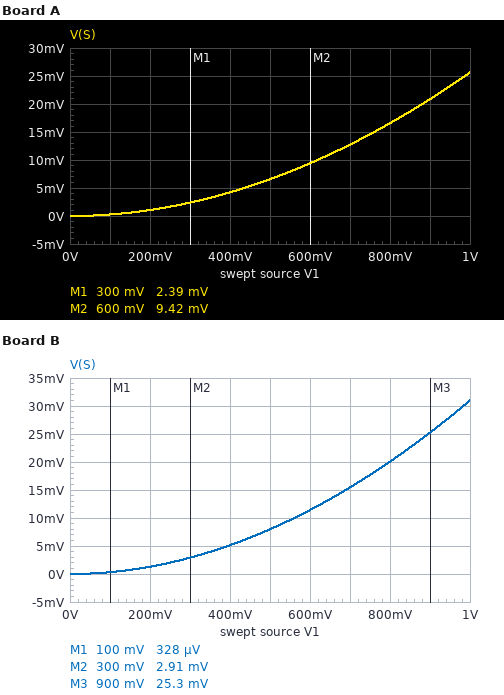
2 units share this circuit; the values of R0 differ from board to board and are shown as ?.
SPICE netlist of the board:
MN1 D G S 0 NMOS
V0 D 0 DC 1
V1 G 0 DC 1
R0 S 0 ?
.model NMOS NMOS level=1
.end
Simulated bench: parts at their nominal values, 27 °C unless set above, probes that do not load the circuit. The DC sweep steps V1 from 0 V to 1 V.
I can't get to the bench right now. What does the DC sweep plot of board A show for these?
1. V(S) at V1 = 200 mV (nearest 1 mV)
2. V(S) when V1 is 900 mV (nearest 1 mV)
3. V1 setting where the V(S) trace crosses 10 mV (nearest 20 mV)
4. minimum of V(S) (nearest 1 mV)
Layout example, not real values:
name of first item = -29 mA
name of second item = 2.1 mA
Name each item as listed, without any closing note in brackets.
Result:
V(S) at V1 = 200 mV = 1 mV
V(S) when V1 is 900 mV = 21 mV
V1 setting where the V(S) trace crosses 10 mV = 620 mV
minimum of V(S) = 0 V
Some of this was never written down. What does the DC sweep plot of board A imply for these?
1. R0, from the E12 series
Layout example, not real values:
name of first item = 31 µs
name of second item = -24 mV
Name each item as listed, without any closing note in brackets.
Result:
R0, from the E12 series = 2.7 kΩ
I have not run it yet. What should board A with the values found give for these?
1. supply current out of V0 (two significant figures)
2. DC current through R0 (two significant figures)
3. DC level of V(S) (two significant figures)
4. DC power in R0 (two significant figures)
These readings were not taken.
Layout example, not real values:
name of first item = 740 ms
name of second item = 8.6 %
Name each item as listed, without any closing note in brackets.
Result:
supply current out of V0 = 9.5 µA
DC current through R0 = 9.5 µA
DC level of V(S) = 26 mV
DC power in R0 = 240 nW
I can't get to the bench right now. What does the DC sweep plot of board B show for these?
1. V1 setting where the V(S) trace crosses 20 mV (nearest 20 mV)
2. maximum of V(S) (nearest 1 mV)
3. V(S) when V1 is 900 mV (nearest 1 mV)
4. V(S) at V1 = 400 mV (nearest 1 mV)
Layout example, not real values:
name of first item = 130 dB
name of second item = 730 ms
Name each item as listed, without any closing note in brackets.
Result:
V1 setting where the V(S) trace crosses 20 mV = 800 mV
maximum of V(S) = 31 mV
V(S) when V1 is 900 mV = 25 mV
V(S) at V1 = 400 mV = 5 mV
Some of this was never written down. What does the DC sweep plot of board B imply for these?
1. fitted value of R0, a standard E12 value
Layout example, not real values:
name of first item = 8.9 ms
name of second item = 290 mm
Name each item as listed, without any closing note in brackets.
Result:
fitted value of R0, a standard E12 value = 3.3 kΩ
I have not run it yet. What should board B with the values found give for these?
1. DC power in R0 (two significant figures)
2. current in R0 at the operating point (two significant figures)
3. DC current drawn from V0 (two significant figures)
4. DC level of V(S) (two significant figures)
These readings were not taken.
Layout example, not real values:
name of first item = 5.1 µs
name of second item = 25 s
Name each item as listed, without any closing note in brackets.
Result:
DC power in R0 = 290 nW
current in R0 at the operating point = 9.4 µA
DC current drawn from V0 = 9.4 µA
DC level of V(S) = 31 mV
